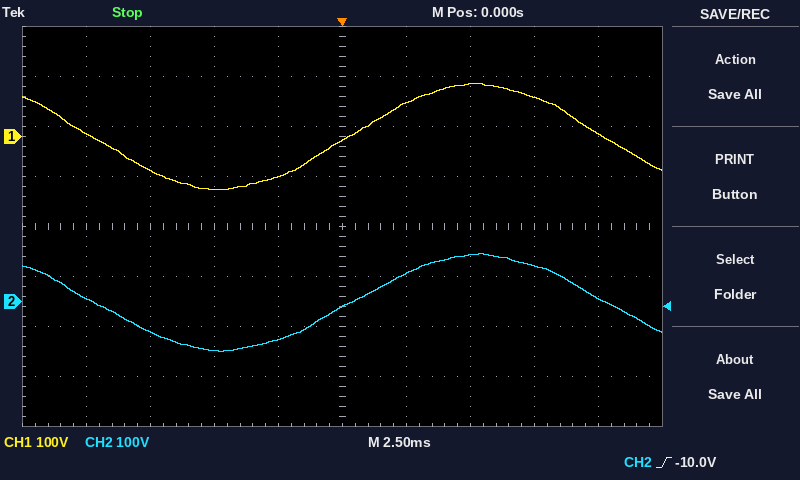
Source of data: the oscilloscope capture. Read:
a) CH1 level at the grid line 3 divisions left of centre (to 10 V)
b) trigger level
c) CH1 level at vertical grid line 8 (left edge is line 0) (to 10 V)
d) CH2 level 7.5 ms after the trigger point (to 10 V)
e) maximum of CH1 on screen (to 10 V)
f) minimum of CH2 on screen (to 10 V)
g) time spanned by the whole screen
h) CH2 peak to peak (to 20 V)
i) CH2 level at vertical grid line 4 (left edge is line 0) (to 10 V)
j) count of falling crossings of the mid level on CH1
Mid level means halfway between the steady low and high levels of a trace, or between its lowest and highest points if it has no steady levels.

-70 V
-10.0 V
80 V
70 V
110 V
-100 V
25 ms
200 V
-80 V
2
